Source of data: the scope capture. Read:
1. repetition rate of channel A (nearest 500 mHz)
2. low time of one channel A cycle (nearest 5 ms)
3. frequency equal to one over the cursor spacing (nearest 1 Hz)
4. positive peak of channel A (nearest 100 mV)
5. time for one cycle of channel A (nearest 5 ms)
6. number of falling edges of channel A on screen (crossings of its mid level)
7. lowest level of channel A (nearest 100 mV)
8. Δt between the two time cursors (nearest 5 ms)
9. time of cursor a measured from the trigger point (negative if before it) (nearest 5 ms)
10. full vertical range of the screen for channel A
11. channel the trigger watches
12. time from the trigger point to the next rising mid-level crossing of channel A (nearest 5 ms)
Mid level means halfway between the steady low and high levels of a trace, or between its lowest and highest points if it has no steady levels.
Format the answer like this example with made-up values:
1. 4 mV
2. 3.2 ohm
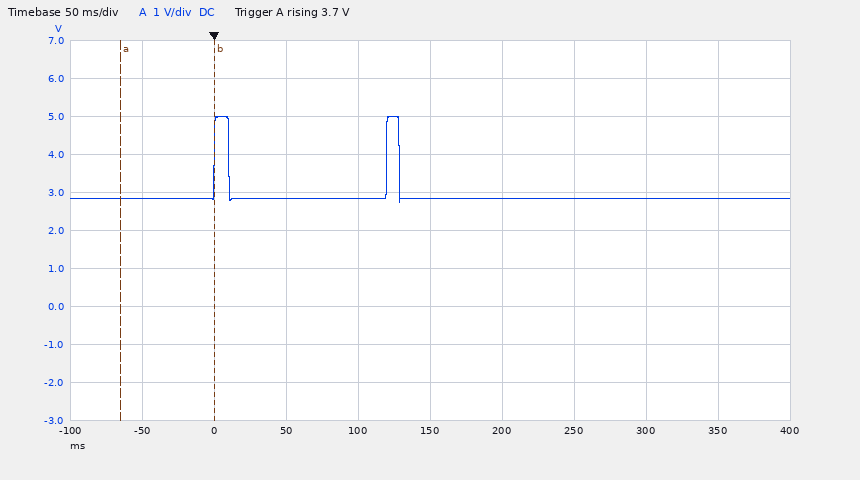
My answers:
1. 8.5 Hz
2. 110 ms
3. 15 Hz
4. 5.0 V
5. 120 ms
6. 2
7. 2.7 V
8. 65 ms
9. -65 ms
10. 10 V
11. channel A
12. 120 ms
